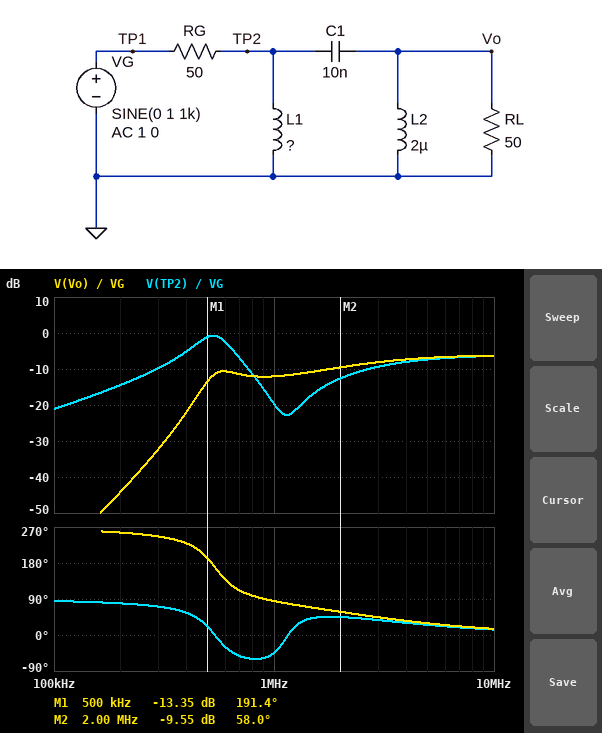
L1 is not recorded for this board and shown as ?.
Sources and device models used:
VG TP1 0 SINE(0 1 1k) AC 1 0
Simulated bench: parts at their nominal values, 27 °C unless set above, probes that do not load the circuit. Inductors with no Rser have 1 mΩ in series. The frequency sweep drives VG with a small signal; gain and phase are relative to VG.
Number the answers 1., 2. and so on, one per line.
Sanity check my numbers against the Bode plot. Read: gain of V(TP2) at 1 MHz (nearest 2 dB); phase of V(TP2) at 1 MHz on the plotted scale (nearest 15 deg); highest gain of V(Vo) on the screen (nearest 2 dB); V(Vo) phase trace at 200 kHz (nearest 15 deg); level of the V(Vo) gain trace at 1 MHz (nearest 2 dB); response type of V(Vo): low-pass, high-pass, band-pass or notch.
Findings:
1. -20 dB
2. -45 deg
3. -6 dB
4. 255 deg
5. -12 dB
6. high-pass
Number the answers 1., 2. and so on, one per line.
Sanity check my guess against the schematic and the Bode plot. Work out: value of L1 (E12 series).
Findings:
1. 6.8 µH
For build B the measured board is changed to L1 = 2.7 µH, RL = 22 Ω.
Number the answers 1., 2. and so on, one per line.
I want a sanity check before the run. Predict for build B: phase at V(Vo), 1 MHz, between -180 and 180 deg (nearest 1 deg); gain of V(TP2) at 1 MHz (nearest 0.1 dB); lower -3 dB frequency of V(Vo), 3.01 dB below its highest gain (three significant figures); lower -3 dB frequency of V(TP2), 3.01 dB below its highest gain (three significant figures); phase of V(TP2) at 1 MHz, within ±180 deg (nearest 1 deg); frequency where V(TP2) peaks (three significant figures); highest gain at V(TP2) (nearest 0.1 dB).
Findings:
1. 92 deg
2. -14.1 dB
3. 675 kHz
4. 605 kHz
5. -18 deg
6. 723 kHz
7. -5.6 dB
